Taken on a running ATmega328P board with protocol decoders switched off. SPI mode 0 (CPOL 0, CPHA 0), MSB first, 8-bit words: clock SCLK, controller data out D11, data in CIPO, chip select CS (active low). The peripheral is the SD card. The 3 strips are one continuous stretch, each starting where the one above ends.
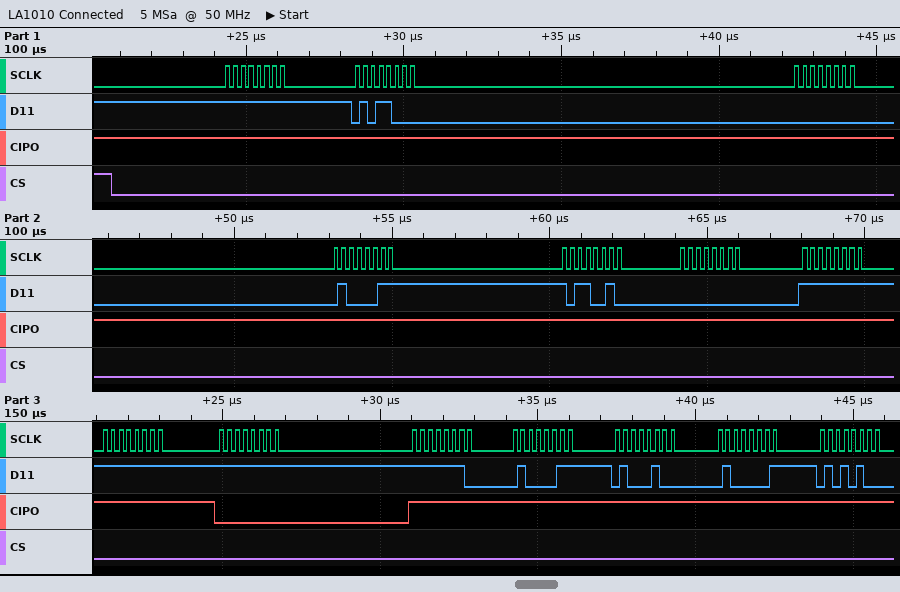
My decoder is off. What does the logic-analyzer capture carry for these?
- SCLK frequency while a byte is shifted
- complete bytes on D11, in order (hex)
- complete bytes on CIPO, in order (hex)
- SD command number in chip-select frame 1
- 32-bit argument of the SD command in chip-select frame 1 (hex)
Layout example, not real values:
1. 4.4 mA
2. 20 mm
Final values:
1. 4 MHz
2. FF 58 00 43 B2 00 FF FF FF FE 43 44 41 54
3. FF FF FF FF FF FF FF FF 00 FF FF FF FF FF
4. CMD24
5. 0x0043B200
